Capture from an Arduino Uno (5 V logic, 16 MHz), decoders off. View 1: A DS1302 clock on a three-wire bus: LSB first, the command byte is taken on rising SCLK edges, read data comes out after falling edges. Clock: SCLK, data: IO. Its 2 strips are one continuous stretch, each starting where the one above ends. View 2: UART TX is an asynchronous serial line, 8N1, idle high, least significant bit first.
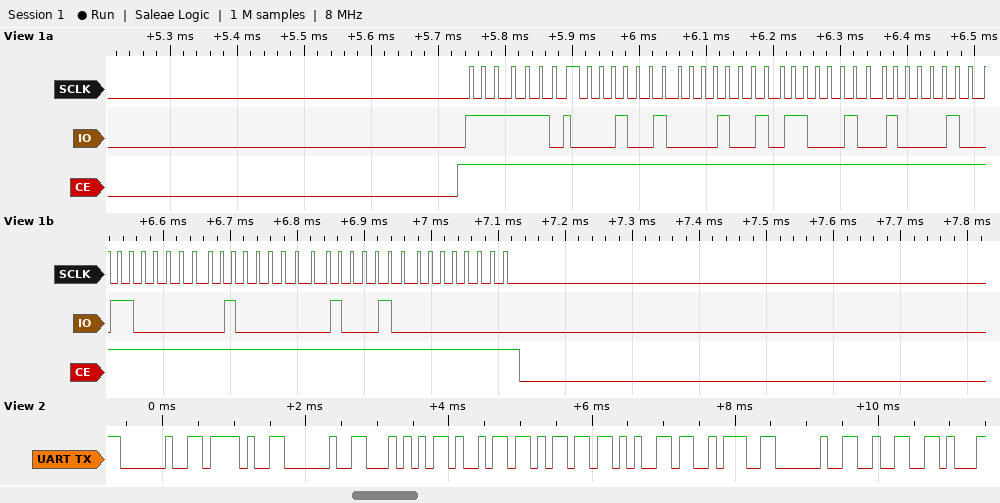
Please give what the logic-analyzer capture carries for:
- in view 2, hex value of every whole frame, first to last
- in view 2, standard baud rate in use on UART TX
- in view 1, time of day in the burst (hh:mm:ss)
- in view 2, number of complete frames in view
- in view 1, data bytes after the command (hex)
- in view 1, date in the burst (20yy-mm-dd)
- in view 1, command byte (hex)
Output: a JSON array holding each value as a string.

["20 2F 20 54 69 6D 65 3A 20 32", "9600 baud", "23:48:48", "10", "48 48 23 21 03 02 22 00", "2022-03-21", "0xBF"]
